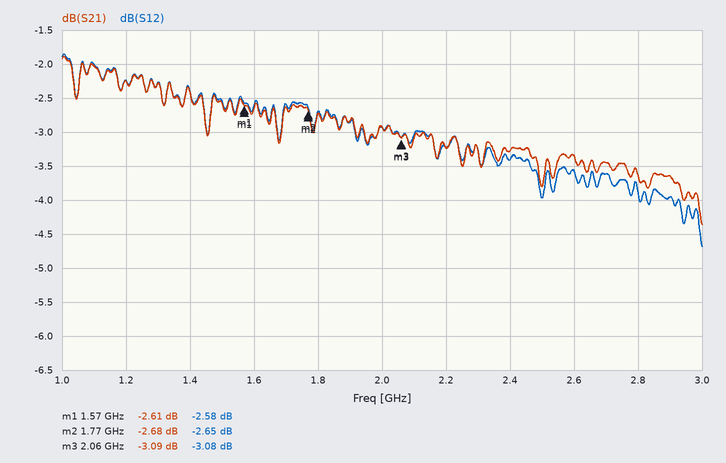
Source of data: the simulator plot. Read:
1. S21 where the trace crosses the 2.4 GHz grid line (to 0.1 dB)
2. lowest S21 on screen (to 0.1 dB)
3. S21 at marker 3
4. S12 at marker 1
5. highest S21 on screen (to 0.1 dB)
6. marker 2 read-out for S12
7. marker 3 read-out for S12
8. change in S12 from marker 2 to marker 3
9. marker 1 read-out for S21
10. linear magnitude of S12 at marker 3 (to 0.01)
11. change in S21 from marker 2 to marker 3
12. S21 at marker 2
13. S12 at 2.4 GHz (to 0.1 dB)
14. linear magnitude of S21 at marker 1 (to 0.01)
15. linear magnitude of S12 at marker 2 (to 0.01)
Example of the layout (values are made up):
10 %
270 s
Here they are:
-3.3 dB
-4.4 dB
-3.09 dB
-2.58 dB
-1.9 dB
-2.65 dB
-3.08 dB
-0.43 dB
-2.61 dB
0.70
-0.41 dB
-2.68 dB
-3.4 dB
0.74
0.74
